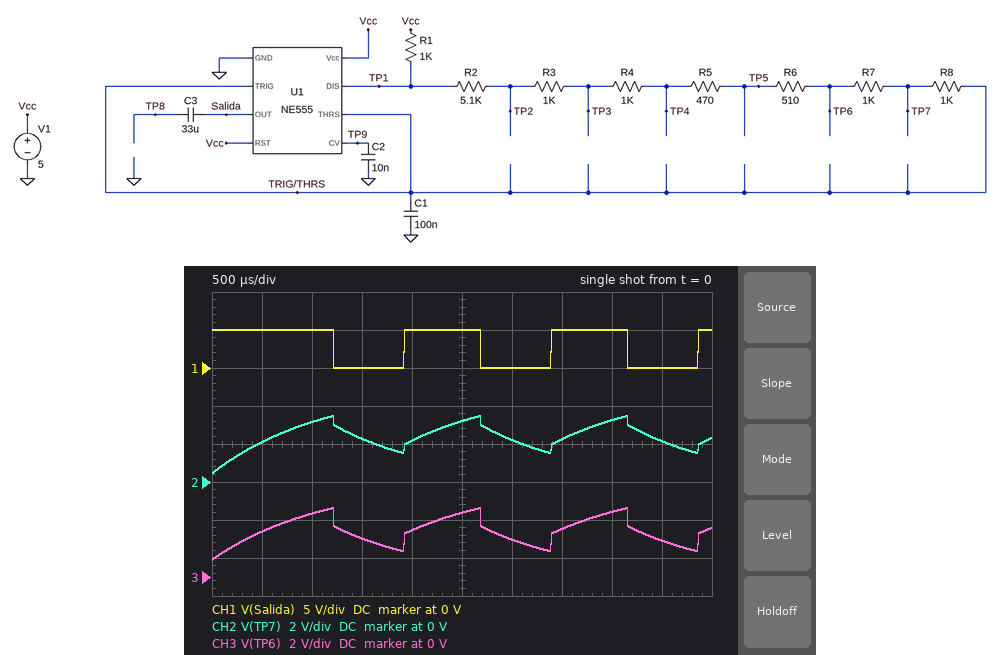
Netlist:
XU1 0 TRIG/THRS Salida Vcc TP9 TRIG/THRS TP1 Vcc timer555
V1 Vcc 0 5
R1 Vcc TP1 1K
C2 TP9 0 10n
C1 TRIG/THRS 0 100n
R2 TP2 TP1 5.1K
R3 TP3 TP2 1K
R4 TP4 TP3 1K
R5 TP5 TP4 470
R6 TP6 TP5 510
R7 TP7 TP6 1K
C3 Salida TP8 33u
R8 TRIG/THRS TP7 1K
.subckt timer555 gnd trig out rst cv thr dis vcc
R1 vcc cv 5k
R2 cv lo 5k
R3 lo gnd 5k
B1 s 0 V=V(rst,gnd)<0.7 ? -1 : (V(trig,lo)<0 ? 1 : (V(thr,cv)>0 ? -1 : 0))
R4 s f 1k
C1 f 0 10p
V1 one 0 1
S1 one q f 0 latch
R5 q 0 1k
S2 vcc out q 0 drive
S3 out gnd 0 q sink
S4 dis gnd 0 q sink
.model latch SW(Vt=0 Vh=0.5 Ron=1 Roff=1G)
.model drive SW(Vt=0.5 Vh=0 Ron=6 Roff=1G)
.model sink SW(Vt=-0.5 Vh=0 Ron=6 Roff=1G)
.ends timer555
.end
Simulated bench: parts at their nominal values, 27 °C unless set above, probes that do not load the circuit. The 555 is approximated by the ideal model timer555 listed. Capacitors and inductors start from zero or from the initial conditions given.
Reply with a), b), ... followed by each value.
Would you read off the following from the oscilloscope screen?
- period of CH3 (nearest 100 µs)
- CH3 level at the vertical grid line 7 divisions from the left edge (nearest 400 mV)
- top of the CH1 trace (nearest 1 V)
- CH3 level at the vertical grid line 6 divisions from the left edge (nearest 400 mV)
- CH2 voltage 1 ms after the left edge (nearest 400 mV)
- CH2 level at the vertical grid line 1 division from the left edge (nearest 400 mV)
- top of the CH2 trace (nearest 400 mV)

a) 1.5 ms
b) 2.4 V
c) 5 V
d) 2.0 V
e) 3.2 V
f) 2.0 V
g) 3.6 V
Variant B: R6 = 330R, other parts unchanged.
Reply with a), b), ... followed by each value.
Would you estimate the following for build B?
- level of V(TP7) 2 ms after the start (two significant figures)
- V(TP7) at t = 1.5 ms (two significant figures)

a) 2.3 V
b) 2.2 V
